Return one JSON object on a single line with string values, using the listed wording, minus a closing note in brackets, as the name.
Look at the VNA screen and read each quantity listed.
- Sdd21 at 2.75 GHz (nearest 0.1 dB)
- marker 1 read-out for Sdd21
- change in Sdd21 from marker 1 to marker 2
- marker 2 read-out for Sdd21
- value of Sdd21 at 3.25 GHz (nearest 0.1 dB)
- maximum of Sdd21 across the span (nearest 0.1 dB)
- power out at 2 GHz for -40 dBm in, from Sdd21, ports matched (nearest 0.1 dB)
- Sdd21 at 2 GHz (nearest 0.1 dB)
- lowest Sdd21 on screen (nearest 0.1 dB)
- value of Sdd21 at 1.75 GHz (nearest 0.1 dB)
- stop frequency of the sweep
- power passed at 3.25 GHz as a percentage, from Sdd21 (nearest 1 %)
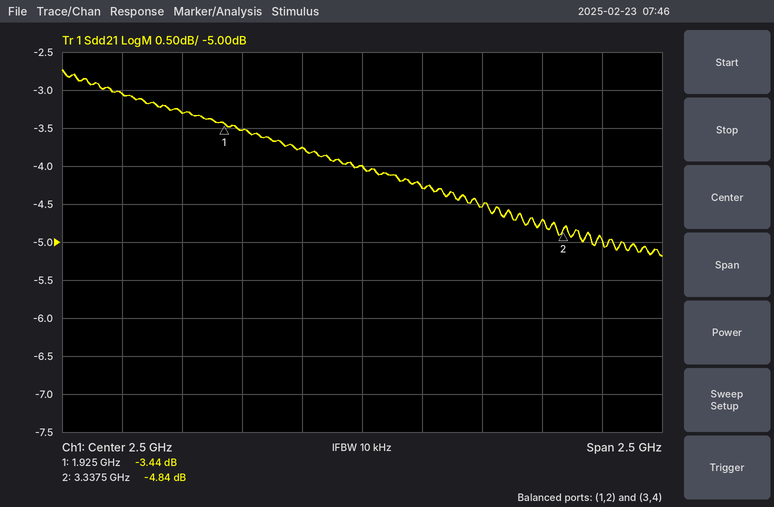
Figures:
{"Sdd21 at 2.75 GHz": "-4.3 dB", "marker 1 read-out for Sdd21": "-3.44 dB", "change in Sdd21 from marker 1 to marker 2": "-1.40 dB", "marker 2 read-out for Sdd21": "-4.84 dB", "value of Sdd21 at 3.25 GHz": "-4.7 dB", "maximum of Sdd21 across the span": "-2.7 dB", "power out at 2 GHz for -40 dBm in, from Sdd21, ports matched": "-43.5 dBm", "Sdd21 at 2 GHz": "-3.5 dB", "lowest Sdd21 on screen": "-5.2 dB", "value of Sdd21 at 1.75 GHz": "-3.3 dB", "stop frequency of the sweep": "3.75 GHz", "power passed at 3.25 GHz as a percentage, from Sdd21": "34 %"}
